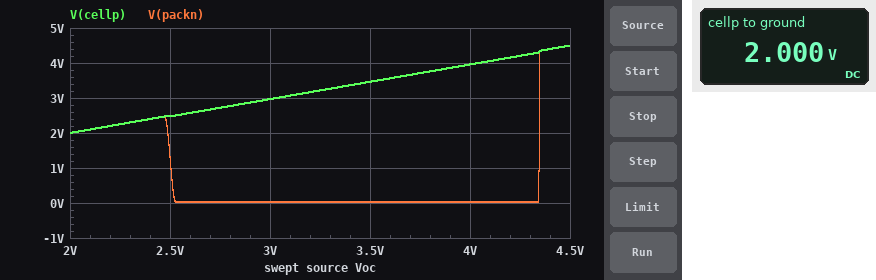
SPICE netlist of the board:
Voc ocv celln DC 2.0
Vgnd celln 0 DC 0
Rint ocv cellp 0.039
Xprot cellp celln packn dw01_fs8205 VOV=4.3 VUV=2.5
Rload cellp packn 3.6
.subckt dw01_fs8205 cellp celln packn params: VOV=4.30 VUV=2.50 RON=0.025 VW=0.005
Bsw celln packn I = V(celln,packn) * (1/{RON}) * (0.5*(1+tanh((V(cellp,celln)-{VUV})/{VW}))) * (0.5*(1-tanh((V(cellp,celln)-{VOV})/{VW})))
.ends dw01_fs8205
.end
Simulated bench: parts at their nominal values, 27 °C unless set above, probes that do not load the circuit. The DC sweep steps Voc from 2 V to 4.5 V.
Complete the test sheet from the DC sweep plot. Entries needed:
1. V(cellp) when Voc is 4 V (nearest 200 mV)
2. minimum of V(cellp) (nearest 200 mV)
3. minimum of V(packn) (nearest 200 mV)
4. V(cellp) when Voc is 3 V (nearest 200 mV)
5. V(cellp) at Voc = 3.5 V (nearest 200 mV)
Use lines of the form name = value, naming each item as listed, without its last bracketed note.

V(cellp) when Voc is 4 V = 4.0 V
minimum of V(cellp) = 2.0 V
minimum of V(packn) = 0 V
V(cellp) when Voc is 3 V = 3.0 V
V(cellp) at Voc = 3.5 V = 3.4 V
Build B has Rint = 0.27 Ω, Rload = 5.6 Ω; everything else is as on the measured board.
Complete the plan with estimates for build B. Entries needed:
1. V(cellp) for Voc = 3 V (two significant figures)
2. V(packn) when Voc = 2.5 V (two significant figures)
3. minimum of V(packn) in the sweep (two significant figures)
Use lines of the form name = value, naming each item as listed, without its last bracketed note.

V(cellp) for Voc = 3 V = 2.9 V
V(packn) when Voc = 2.5 V = 2.1 V
minimum of V(packn) in the sweep = 11 mV
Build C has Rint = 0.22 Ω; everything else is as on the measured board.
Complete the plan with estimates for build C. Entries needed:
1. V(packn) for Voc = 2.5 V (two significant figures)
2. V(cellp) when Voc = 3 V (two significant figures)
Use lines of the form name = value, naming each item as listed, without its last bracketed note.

V(packn) for Voc = 2.5 V = 2.2 V
V(cellp) when Voc = 3 V = 2.8 V
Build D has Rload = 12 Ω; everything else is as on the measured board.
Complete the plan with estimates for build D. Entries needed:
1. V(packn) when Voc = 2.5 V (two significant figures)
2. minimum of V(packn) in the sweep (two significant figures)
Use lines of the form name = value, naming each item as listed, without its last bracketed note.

V(packn) when Voc = 2.5 V = 110 mV
minimum of V(packn) in the sweep = 5.2 mV
